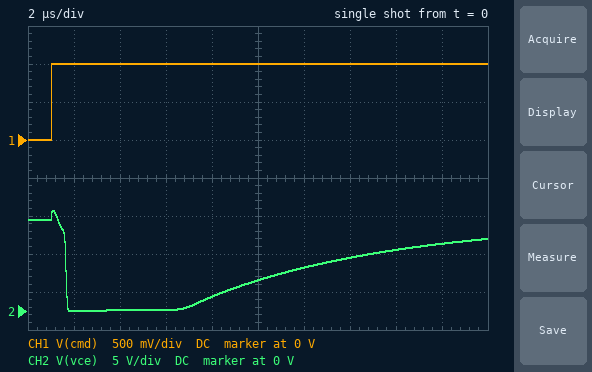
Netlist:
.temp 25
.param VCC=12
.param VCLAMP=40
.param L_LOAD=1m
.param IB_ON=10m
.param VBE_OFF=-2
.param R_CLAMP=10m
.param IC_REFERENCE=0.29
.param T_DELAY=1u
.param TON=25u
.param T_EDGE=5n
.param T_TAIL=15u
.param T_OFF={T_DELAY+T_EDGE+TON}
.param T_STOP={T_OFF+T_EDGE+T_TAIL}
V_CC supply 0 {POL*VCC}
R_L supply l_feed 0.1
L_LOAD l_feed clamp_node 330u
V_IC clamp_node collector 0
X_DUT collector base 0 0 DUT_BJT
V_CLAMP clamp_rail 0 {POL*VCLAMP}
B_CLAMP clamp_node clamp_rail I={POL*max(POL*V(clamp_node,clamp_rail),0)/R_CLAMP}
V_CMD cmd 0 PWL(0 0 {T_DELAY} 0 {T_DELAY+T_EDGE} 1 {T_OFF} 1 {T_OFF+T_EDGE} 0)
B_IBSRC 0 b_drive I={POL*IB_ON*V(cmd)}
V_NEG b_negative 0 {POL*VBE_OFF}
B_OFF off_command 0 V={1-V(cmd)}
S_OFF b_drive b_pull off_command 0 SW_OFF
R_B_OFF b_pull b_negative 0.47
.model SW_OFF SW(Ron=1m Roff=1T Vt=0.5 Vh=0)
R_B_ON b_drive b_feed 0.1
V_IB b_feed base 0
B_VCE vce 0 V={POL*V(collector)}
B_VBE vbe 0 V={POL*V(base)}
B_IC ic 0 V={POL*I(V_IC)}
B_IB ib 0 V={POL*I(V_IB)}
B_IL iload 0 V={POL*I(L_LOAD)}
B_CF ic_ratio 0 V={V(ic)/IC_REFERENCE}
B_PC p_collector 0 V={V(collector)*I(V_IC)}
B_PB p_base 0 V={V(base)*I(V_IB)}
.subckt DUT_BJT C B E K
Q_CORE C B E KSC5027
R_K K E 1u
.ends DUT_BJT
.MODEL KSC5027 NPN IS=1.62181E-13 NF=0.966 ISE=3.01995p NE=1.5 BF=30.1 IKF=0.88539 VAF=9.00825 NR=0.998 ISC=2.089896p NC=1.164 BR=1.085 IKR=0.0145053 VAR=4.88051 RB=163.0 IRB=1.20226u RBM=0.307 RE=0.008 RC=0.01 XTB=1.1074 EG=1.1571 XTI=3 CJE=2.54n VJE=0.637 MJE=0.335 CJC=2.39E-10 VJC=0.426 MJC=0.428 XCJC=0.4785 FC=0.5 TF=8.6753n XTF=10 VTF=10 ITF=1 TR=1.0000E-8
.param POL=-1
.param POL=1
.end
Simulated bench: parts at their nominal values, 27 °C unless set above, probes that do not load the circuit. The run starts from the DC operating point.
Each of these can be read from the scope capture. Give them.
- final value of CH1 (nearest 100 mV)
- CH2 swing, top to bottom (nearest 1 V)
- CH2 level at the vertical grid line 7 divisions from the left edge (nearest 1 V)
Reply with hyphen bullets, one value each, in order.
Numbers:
- 1.0 V
- 13 V
- 7 V
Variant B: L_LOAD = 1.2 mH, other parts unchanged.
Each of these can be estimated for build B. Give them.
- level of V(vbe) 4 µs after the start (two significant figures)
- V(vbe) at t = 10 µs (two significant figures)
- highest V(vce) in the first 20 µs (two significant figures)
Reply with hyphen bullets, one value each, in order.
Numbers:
- 690 mV
- 710 mV
- 14 V
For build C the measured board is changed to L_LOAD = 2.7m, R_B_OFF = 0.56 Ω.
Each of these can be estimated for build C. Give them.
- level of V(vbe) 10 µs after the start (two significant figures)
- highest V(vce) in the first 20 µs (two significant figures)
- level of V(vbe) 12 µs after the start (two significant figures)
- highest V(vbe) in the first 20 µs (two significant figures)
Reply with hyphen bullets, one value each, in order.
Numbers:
- 690 mV
- 14 V
- 700 mV
- 1.9 V
